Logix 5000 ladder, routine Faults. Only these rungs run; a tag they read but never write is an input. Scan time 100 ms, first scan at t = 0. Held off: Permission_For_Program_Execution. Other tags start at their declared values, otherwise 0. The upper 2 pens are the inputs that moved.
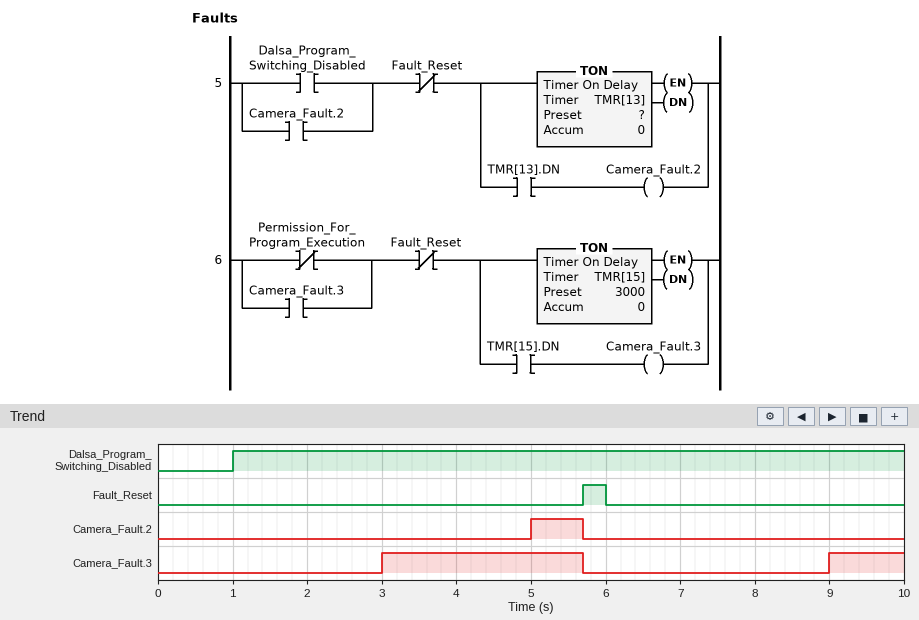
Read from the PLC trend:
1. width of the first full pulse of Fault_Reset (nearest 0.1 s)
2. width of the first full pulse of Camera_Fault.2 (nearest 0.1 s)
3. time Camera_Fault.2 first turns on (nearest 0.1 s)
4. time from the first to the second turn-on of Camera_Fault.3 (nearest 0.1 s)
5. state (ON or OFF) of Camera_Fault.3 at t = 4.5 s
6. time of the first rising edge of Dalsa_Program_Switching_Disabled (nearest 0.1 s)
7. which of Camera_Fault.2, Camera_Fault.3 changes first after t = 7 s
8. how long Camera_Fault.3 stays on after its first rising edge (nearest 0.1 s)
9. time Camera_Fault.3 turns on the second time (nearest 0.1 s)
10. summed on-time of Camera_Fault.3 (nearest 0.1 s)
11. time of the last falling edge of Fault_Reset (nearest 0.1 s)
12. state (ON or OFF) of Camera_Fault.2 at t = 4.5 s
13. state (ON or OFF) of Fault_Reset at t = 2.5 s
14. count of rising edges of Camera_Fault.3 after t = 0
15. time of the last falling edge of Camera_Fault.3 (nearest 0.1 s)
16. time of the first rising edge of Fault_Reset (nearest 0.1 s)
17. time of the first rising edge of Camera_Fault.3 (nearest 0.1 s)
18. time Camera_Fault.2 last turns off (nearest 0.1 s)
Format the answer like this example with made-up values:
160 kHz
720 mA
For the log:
0.3 s
0.7 s
5.0 s
6.0 s
ON
1.0 s
Camera_Fault.3
2.7 s
9.0 s
3.7 s
6.0 s
OFF
OFF
2
5.7 s
5.7 s
3.0 s
5.7 s
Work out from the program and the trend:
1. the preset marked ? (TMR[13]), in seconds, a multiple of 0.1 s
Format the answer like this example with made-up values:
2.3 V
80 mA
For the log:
4.0 s
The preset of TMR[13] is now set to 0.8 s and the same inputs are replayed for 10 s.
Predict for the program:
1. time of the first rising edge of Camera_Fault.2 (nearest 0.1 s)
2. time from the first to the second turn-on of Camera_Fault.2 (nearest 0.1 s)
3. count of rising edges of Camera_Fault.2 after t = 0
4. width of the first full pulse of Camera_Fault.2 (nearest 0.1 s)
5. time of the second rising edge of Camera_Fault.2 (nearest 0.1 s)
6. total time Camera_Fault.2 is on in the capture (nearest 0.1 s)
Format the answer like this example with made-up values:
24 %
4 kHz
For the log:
1.8 s
5.0 s
2
3.9 s
6.8 s
7.1 s
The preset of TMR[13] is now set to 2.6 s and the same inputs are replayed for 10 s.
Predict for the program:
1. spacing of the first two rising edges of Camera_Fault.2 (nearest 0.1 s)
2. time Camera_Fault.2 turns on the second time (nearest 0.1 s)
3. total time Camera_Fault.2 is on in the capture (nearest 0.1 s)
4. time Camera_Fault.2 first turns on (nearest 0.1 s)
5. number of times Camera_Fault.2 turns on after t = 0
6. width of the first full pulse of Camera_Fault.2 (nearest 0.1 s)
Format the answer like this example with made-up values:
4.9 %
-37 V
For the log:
5.0 s
8.6 s
3.5 s
3.6 s
2
2.1 s
